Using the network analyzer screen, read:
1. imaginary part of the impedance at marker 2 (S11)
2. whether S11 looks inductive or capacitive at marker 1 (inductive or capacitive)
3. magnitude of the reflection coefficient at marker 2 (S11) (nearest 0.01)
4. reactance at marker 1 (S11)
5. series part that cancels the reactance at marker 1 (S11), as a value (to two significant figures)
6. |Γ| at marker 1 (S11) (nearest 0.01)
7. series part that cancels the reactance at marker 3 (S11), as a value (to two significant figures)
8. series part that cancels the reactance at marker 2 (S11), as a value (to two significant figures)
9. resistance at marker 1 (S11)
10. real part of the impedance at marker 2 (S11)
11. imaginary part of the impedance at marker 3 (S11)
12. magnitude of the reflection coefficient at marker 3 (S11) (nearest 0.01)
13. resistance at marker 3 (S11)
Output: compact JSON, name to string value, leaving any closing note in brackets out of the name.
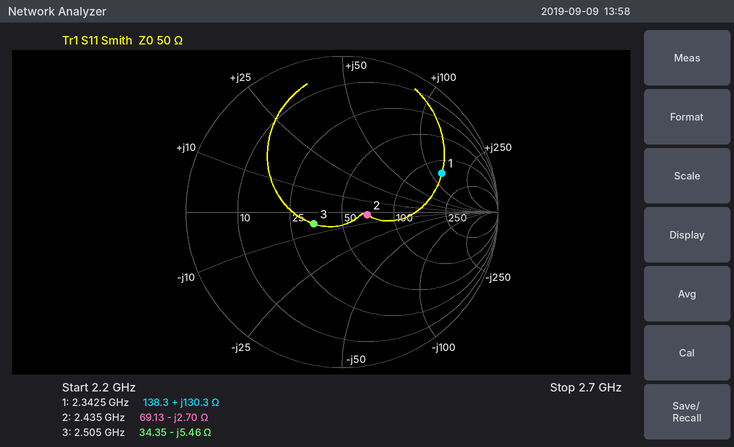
{"imaginary part of the impedance at marker 2": "-2.70 Ω", "whether S11 looks inductive or capacitive at marker 1": "inductive", "magnitude of the reflection coefficient at marker 2 (S11)": "0.16", "reactance at marker 1": "+130.3 Ω", "series part that cancels the reactance at marker 1 (S11), as a value": "520 fF", "|Γ| at marker 1 (S11)": "0.69", "series part that cancels the reactance at marker 3 (S11), as a value": "350 pH", "series part that cancels the reactance at marker 2 (S11), as a value": "180 pH", "resistance at marker 1": "138.3 Ω", "real part of the impedance at marker 2": "69.13 Ω", "imaginary part of the impedance at marker 3": "-5.46 Ω", "magnitude of the reflection coefficient at marker 3 (S11)": "0.20", "resistance at marker 3": "34.35 Ω"}
